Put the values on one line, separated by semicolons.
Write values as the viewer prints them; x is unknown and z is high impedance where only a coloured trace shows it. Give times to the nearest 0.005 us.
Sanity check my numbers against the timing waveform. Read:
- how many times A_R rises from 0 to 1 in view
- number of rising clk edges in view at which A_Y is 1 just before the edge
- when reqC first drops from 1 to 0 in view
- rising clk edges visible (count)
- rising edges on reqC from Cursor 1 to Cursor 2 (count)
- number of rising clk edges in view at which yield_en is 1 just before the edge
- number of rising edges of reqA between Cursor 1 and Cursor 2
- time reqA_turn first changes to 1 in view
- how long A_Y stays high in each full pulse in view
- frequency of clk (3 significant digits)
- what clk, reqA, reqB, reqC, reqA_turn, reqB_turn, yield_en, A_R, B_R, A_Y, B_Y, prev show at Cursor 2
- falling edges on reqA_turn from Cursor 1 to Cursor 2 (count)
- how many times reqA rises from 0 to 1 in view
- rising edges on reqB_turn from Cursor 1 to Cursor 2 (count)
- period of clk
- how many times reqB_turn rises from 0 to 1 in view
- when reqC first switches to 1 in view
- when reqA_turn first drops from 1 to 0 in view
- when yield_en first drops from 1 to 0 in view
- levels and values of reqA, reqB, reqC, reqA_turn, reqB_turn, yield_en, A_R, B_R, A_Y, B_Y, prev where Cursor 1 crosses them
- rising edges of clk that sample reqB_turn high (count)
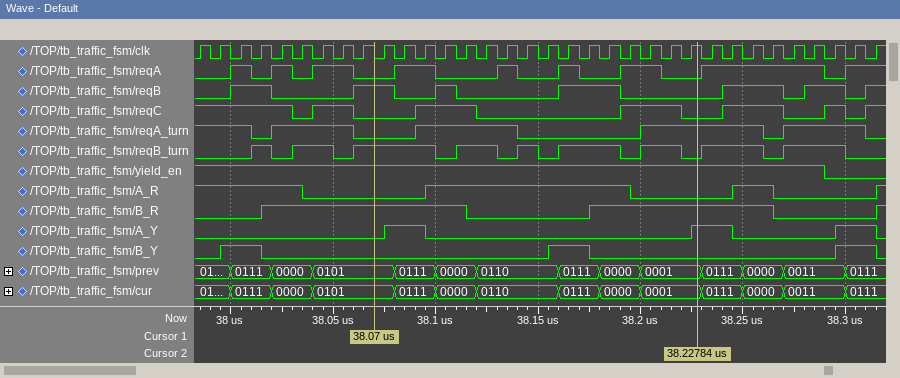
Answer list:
3; 6; 38.03 us; 34; 2; 31; 4; 38.02 us; 0.02 us, 0.02 us, 0.02 us; 100 MHz; clk=1, reqA=0, reqB=0, reqC=0, reqA_turn=1, reqB_turn=0, yield_en=1, A_R=0, B_R=1, A_Y=1, B_Y=0, prev=0001; 1; 9; 4; 0.01 us; 9; 38.04 us; 38.01 us; 38.29 us; reqA=0, reqB=1, reqC=0, reqA_turn=0, reqB_turn=1, yield_en=1, A_R=0, B_R=1, A_Y=0, B_Y=0, prev=0101; 21
